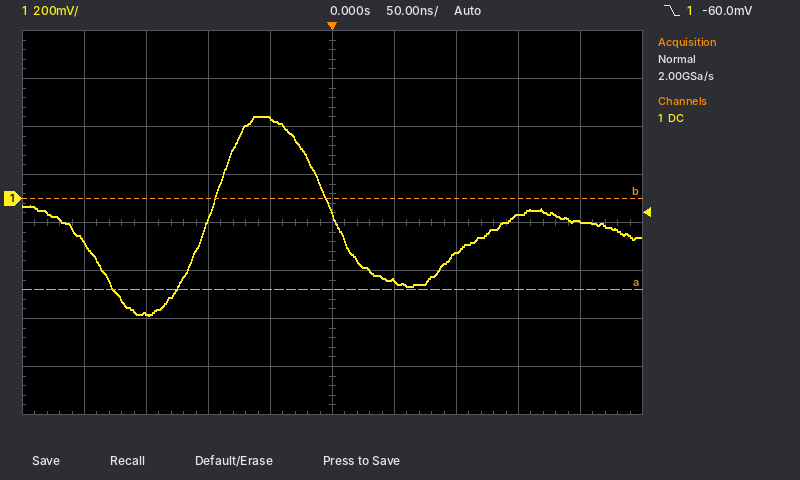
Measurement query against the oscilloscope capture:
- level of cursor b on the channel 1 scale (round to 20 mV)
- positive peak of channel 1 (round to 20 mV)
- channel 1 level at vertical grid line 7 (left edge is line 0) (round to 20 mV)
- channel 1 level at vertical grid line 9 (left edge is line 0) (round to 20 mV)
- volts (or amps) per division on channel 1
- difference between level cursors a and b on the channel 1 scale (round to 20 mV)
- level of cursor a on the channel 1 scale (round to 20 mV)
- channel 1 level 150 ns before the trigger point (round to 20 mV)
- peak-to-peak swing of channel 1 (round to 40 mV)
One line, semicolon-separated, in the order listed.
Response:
0 mV; 340 mV; -220 mV; -100 mV; 200 mV; 380 mV; -380 mV; -480 mV; 840 mV
